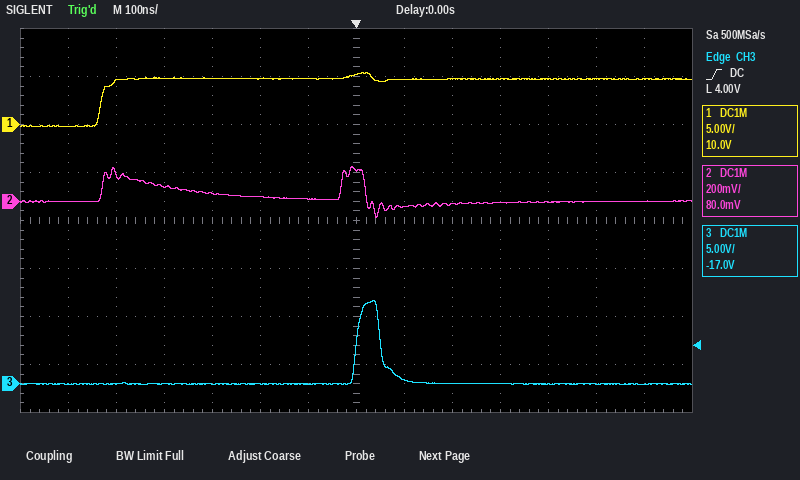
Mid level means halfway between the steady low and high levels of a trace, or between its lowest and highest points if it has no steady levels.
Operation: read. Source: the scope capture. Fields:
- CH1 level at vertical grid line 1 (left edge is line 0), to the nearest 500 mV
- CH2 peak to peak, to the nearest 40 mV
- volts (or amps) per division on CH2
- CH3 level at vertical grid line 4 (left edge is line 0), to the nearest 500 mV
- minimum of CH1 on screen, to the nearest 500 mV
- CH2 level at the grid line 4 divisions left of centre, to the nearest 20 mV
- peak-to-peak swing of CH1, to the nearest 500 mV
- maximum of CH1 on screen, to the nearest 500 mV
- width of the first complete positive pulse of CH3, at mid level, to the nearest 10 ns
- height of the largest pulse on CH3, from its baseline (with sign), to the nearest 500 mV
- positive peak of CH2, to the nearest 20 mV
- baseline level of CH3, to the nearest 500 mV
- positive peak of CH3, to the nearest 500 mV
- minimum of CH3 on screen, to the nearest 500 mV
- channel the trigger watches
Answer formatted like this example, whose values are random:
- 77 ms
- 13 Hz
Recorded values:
- 0.0 V
- 200 mV
- 200 mV
- 0.0 V
- 0.0 V
- 60 mV
- 5.5 V
- 5.5 V
- 50 ns
- +8.5 V
- 140 mV
- 0.0 V
- 8.5 V
- 0.0 V
- CH3
